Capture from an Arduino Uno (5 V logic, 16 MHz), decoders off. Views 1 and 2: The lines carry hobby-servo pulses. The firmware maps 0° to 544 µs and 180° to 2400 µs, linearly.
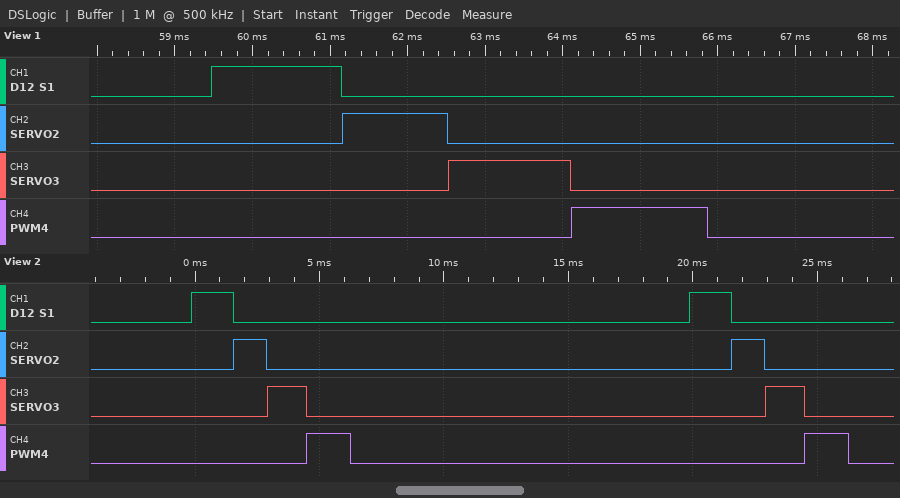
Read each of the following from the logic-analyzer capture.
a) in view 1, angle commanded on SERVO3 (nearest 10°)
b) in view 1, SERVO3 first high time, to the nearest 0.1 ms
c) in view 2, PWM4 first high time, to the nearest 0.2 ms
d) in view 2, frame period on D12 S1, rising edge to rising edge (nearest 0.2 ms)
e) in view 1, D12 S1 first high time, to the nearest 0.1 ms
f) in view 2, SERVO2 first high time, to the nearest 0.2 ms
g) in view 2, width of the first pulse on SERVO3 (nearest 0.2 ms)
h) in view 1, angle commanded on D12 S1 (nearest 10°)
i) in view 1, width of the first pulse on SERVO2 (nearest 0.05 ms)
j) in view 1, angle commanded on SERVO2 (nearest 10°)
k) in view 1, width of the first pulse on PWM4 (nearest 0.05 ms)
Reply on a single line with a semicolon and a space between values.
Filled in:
100°; 1.6 ms; 1.8 ms; 20.0 ms; 1.7 ms; 1.4 ms; 1.6 ms; 110°; 1.35 ms; 80°; 1.75 ms
